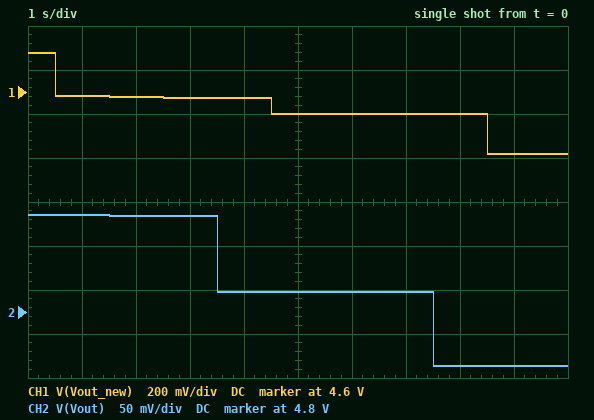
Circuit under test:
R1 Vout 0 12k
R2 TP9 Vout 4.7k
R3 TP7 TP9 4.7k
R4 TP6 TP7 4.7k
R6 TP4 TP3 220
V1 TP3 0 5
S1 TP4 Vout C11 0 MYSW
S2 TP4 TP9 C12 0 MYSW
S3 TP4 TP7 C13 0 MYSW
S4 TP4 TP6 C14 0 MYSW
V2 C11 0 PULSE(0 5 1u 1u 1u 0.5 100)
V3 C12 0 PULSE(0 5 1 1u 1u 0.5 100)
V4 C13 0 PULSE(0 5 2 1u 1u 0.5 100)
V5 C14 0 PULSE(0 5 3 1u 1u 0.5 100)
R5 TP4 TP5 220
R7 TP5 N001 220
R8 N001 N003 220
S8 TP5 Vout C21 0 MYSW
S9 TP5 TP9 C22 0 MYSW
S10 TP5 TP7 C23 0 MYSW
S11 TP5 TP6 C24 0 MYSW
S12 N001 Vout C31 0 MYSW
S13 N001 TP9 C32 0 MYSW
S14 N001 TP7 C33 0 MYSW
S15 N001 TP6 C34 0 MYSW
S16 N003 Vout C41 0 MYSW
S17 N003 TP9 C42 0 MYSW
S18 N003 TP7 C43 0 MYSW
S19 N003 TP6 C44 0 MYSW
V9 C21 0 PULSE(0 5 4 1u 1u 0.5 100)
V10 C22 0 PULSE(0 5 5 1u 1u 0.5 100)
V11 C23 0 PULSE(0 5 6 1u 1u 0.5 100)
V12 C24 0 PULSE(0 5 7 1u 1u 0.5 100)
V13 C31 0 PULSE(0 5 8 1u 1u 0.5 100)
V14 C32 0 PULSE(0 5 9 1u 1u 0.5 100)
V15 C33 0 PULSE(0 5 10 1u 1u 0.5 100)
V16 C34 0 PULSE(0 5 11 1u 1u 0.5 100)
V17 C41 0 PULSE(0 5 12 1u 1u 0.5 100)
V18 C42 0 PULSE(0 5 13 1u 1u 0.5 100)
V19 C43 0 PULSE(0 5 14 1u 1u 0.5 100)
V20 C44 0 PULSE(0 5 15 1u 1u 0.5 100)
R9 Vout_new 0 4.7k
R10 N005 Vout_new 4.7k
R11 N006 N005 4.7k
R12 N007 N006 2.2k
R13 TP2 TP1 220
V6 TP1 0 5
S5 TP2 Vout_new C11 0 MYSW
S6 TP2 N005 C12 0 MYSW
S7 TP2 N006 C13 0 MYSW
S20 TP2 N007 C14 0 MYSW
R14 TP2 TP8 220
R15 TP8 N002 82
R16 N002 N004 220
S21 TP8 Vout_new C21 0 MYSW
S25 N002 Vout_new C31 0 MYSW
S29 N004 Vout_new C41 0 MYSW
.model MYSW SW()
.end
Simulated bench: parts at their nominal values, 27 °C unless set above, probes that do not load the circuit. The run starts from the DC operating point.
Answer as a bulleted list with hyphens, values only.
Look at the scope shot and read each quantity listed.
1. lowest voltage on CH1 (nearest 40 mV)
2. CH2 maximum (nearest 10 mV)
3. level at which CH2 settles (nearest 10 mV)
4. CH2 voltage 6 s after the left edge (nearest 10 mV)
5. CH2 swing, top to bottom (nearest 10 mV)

- 4.32 V
- 4.91 V
- 4.74 V
- 4.82 V
- 170 mV
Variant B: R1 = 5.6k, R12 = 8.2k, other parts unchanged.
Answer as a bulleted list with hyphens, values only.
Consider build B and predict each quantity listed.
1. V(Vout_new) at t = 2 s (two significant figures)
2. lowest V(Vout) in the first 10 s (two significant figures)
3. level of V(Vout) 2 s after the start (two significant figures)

- 4.6 V
- 4.5 V
- 4.8 V
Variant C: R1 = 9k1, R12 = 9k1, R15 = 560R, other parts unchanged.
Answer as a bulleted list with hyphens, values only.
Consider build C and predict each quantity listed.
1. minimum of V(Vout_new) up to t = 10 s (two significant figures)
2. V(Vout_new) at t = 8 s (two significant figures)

- 4.0 V
- 4.1 V
